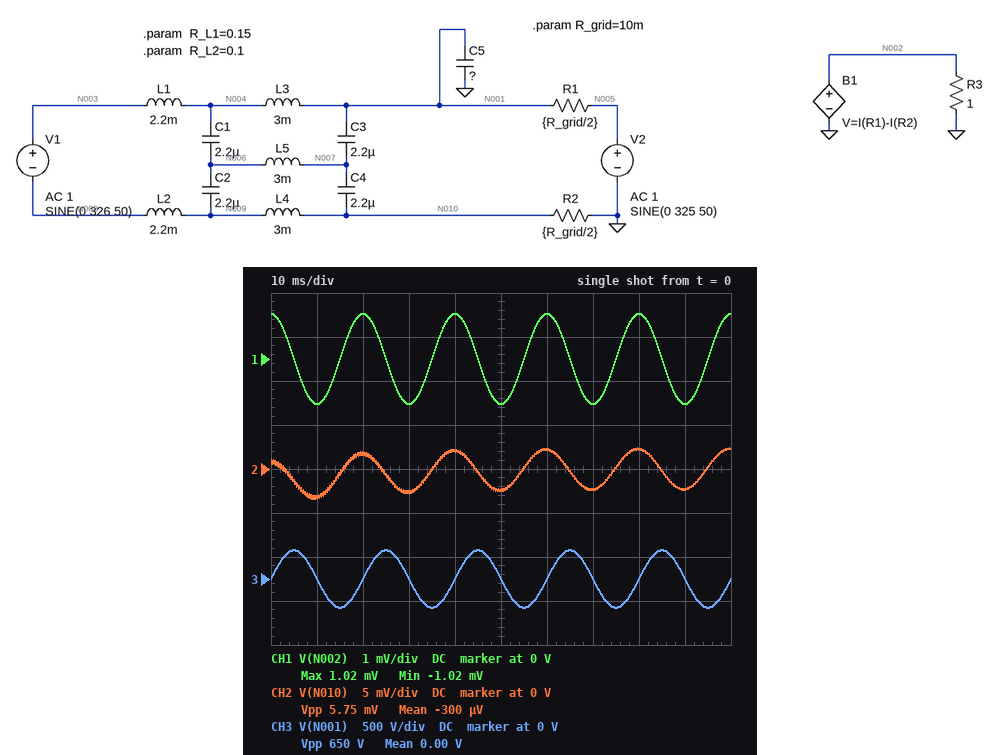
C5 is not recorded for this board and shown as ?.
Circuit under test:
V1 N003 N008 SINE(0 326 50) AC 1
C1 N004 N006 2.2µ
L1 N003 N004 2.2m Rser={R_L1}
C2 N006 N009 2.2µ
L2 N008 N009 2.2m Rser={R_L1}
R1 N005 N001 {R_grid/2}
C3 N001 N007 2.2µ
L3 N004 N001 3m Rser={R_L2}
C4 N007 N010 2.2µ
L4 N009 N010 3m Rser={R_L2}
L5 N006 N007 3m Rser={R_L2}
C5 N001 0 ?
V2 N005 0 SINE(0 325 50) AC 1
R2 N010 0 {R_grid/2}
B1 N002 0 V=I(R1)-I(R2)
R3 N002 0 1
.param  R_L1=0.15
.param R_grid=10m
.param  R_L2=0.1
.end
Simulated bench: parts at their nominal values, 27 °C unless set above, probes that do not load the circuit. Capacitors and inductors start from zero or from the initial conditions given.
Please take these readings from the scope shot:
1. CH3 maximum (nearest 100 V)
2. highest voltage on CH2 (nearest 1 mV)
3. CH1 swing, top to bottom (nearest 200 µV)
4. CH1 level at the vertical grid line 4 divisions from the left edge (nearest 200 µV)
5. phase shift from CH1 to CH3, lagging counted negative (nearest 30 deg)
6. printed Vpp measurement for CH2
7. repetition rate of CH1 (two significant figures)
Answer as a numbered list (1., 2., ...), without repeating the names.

1. 300 V
2. 2 mV
3. 2.0 mV
4. 1.0 mV
5. -90 deg
6. 5.75 mV
7. 50 Hz
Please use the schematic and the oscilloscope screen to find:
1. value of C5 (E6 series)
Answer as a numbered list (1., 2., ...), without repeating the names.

1. 10 nF
